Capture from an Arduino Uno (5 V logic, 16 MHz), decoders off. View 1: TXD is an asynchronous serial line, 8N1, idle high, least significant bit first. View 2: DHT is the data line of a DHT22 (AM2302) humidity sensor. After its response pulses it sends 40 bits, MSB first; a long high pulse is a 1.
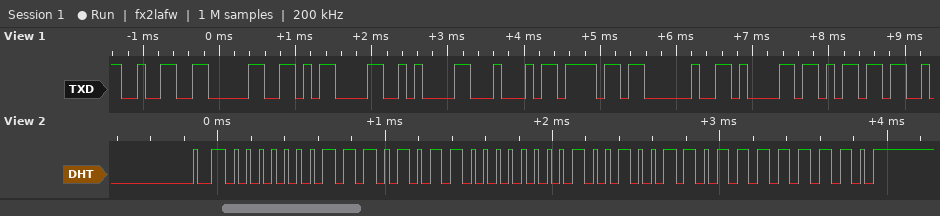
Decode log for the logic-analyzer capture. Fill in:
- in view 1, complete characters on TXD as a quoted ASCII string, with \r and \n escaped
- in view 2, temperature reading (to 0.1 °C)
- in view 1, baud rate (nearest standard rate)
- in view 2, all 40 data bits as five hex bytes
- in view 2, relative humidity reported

"20\r\nDo am"
29.4 °C
9600 baud
01 D6 01 26 FE
47.0 %
